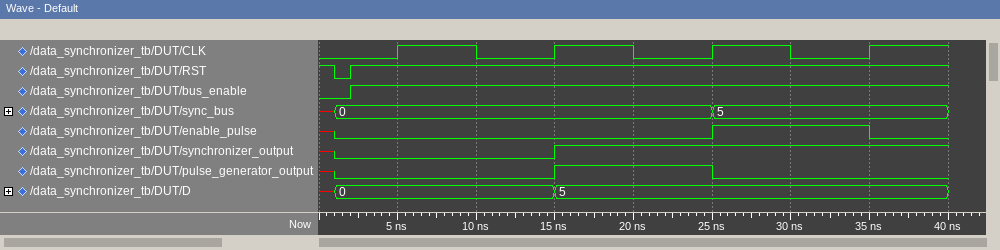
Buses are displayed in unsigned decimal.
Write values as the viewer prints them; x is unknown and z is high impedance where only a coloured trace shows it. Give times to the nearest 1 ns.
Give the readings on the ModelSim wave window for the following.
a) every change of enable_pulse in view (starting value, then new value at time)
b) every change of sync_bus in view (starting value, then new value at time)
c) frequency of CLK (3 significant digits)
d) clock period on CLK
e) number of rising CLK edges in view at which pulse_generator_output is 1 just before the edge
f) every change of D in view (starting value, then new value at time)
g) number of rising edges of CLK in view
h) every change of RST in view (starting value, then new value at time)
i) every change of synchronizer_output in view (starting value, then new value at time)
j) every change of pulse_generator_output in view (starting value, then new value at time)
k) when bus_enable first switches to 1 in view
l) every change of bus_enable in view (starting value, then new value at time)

x, 0 at 1 ns, 1 at 25 ns, 0 at 35 ns
x, 0 at 1 ns, 5 at 25 ns
100 MHz
10 ns
1
x, 0 at 1 ns, 5 at 15 ns
4
1, 0 at 1 ns, 1 at 2 ns
x, 0 at 1 ns, 1 at 15 ns
x, 0 at 1 ns, 1 at 15 ns, 0 at 25 ns
2 ns
0, 1 at 2 ns
